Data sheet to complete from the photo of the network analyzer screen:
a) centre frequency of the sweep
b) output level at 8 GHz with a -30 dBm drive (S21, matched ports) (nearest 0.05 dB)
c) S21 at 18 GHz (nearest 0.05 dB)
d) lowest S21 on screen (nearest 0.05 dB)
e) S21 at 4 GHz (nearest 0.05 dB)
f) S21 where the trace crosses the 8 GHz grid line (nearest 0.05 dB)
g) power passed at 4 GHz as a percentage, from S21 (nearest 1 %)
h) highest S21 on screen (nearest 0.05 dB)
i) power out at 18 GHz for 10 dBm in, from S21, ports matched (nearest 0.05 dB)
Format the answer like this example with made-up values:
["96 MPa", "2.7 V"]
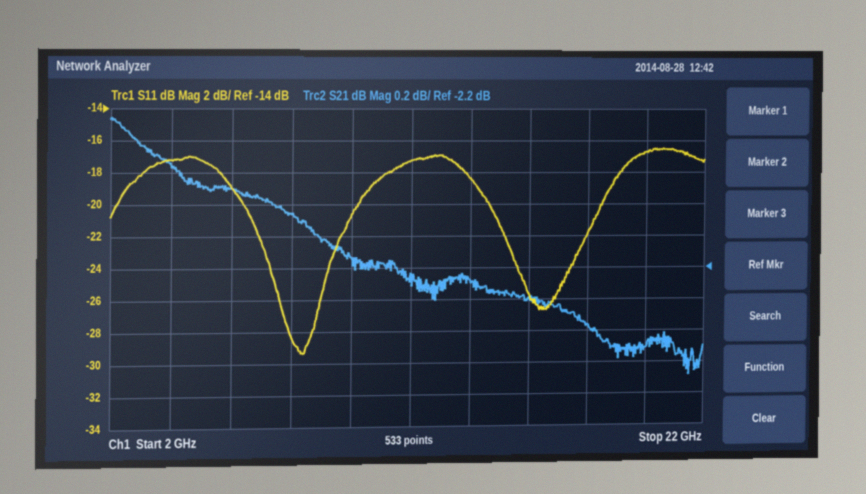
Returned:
["12 GHz", "-31.85 dBm", "-2.55 dB", "-2.90 dB", "-1.55 dB", "-1.85 dB", "70 %", "-1.25 dB", "7.45 dBm"]
